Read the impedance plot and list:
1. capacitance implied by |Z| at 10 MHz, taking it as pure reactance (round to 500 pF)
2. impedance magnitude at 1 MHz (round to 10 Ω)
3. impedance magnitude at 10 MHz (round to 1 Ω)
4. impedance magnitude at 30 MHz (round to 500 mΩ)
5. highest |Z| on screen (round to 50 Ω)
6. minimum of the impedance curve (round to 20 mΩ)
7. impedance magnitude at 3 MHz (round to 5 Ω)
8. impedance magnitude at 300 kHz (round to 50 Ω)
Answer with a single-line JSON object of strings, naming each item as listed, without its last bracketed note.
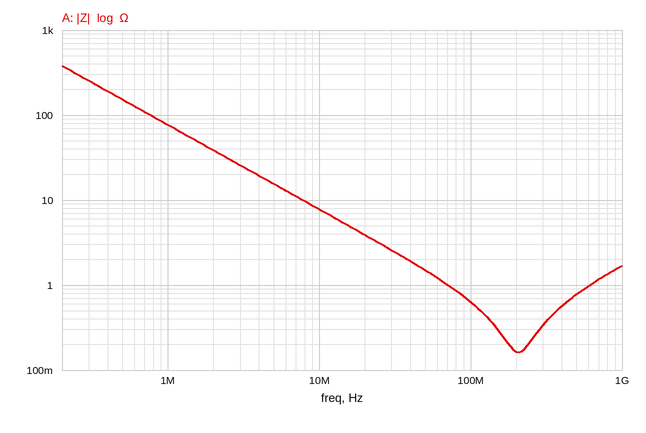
{"capacitance implied by |Z| at 10 MHz, taking it as pure reactance": "2.0 nF", "impedance magnitude at 1 MHz": "80 Ω", "impedance magnitude at 10 MHz": "8 Ω", "impedance magnitude at 30 MHz": "2.5 Ω", "highest |Z| on screen": "400 Ω", "minimum of the impedance curve": "160 mΩ", "impedance magnitude at 3 MHz": "25 Ω", "impedance magnitude at 300 kHz": "250 Ω"}
